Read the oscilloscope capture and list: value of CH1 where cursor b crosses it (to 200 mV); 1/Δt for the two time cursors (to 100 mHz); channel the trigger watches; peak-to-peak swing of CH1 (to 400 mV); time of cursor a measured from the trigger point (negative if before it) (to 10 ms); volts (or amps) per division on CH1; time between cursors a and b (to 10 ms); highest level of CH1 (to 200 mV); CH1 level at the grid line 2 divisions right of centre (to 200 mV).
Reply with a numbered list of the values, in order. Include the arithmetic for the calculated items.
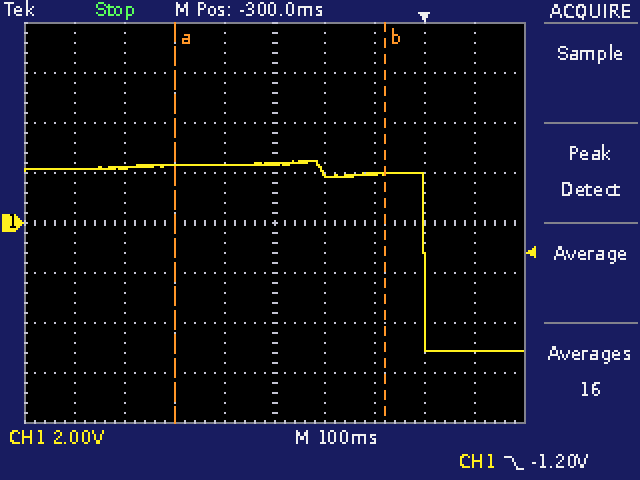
1. 2.0 V
2. 1 / 420 ms ≈ 2.4 Hz
3. CH1
4. 7.6 V
5. -500 ms
6. 2 V
7. 420 ms
8. 2.4 V
9. 2.0 V
